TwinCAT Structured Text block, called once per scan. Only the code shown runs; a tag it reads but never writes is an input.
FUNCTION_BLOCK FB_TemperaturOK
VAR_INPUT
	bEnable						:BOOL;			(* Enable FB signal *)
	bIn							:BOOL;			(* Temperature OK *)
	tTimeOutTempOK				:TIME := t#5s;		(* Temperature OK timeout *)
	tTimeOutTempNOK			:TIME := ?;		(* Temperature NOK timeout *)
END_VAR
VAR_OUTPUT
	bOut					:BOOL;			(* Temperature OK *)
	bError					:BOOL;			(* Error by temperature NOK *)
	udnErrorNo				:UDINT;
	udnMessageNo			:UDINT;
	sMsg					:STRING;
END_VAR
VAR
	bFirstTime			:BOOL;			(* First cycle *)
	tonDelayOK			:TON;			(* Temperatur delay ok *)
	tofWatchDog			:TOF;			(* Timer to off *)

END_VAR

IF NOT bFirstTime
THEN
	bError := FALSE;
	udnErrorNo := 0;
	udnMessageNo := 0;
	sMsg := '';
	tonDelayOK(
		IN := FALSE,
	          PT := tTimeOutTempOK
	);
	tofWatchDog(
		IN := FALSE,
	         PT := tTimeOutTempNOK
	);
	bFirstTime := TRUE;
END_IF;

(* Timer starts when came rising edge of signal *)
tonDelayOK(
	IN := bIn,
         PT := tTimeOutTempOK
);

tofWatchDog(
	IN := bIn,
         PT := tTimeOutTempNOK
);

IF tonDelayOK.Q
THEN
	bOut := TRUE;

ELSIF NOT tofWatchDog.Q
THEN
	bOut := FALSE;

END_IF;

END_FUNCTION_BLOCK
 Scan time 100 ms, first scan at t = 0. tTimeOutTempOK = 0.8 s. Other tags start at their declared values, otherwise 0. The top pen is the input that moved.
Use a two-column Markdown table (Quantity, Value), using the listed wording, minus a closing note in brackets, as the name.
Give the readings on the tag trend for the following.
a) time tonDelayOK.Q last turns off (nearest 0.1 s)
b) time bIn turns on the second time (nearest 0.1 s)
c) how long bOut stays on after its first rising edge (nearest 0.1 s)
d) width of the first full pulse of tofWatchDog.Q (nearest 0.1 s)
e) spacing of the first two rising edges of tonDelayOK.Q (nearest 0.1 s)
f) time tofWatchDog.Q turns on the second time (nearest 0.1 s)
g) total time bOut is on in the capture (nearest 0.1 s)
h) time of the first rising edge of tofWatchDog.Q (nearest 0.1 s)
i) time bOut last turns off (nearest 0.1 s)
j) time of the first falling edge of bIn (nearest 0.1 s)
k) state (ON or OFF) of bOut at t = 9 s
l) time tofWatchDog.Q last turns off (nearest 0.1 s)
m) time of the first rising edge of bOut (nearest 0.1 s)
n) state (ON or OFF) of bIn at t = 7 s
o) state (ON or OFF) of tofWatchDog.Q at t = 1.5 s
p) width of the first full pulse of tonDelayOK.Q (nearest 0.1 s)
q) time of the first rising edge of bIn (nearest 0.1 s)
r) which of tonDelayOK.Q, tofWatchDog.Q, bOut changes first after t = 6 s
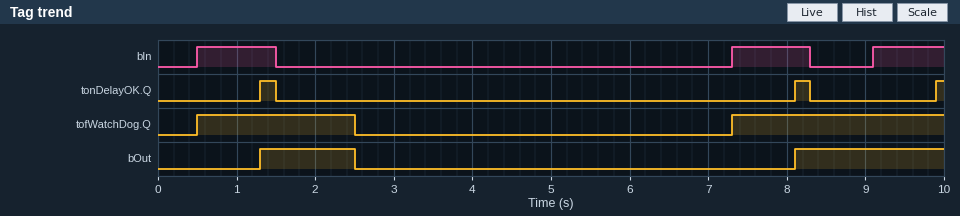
| Quantity | Value |
|---|---|
| time tonDelayOK.Q last turns off | 8.3 s |
| time bIn turns on the second time | 7.3 s |
| how long bOut stays on after its first rising edge | 1.2 s |
| width of the first full pulse of tofWatchDog.Q | 2.0 s |
| spacing of the first two rising edges of tonDelayOK.Q | 6.8 s |
| time tofWatchDog.Q turns on the second time | 7.3 s |
| total time bOut is on in the capture | 3.1 s |
| time of the first rising edge of tofWatchDog.Q | 0.5 s |
| time bOut last turns off | 2.5 s |
| time of the first falling edge of bIn | 1.5 s |
| state (ON or OFF) of bOut at t = 9 s | ON |
| time tofWatchDog.Q last turns off | 2.5 s |
| time of the first rising edge of bOut | 1.3 s |
| state (ON or OFF) of bIn at t = 7 s | OFF |
| state (ON or OFF) of tofWatchDog.Q at t = 1.5 s | ON |
| width of the first full pulse of tonDelayOK.Q | 0.2 s |
| time of the first rising edge of bIn | 0.5 s |
| which of tonDelayOK.Q, tofWatchDog.Q, bOut changes first after t = 6 s | tofWatchDog.Q |
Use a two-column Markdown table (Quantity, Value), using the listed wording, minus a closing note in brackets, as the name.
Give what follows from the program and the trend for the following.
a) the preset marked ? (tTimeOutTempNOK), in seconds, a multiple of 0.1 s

| Quantity | Value |
|---|---|
| the preset marked ? (tTimeOutTempNOK), in seconds, a multiple of 0.1 s | 1.0 s |
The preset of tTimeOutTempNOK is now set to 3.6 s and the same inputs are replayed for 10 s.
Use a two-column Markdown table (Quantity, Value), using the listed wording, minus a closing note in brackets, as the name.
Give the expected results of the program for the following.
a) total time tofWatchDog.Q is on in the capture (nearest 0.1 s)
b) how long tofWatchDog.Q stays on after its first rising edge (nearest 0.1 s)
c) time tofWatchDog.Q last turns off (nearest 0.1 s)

| Quantity | Value |
|---|---|
| total time tofWatchDog.Q is on in the capture | 7.3 s |
| how long tofWatchDog.Q stays on after its first rising edge | 4.6 s |
| time tofWatchDog.Q last turns off | 5.1 s |
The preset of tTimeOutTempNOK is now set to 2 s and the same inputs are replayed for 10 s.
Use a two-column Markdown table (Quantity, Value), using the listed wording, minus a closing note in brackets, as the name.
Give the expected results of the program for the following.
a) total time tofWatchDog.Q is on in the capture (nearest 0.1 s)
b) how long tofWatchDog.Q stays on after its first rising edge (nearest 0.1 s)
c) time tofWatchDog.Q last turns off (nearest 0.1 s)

| Quantity | Value |
|---|---|
| total time tofWatchDog.Q is on in the capture | 5.7 s |
| how long tofWatchDog.Q stays on after its first rising edge | 3.0 s |
| time tofWatchDog.Q last turns off | 3.5 s |
